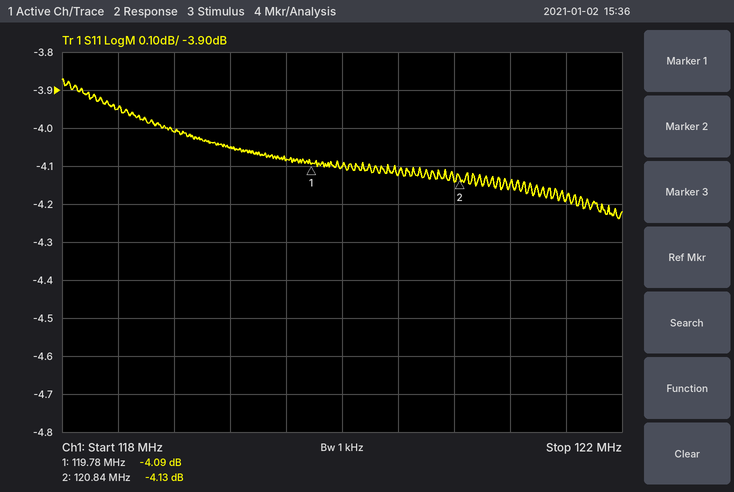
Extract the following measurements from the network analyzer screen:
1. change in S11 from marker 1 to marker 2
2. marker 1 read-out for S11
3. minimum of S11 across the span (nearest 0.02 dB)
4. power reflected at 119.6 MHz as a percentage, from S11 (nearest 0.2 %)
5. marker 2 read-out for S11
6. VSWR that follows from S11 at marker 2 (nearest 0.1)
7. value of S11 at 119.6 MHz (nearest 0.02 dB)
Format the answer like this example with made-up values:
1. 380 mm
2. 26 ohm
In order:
1. -0.04 dB
2. -4.09 dB
3. -4.24 dB
4. 39.0 %
5. -4.13 dB
6. 4.3
7. -4.08 dB
